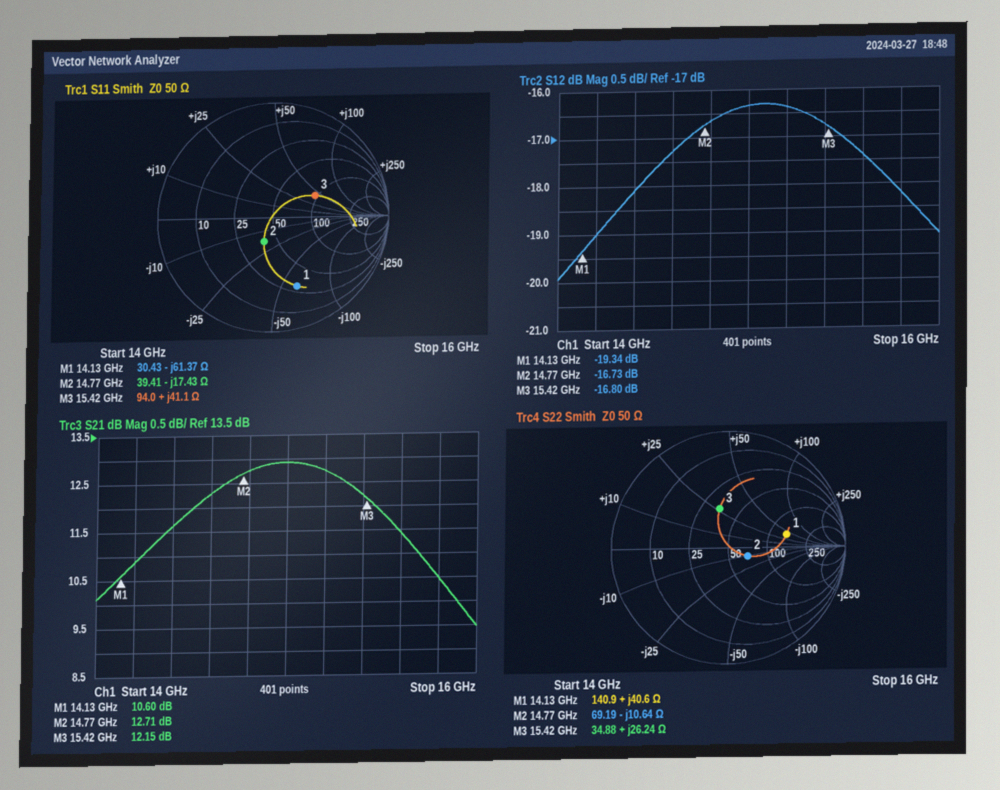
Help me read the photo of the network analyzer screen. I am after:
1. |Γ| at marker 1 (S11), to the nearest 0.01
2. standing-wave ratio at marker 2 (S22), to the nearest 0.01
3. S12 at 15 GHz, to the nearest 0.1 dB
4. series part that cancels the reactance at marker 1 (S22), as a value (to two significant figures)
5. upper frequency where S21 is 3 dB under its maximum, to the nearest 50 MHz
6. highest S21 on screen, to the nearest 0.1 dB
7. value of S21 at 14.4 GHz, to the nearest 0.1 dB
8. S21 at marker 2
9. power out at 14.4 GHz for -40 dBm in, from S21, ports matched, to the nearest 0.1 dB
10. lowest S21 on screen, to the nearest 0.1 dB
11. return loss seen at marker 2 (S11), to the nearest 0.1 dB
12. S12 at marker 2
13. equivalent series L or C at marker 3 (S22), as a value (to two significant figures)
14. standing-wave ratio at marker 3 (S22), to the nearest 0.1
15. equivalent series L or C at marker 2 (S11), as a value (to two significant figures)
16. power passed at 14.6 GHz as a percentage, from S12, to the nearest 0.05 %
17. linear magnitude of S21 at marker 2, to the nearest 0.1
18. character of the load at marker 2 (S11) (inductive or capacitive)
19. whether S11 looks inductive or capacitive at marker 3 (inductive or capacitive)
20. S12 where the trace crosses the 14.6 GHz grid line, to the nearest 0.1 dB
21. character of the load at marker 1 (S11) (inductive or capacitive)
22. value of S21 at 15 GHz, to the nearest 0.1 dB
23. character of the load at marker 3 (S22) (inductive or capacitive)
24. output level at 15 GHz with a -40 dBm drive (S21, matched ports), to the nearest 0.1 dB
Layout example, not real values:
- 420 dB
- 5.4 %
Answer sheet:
- 0.64
- 1.45
- -16.3 dB
- 280 fF
- 15.90 GHz
- 12.9 dB
- 11.6 dB
- 12.71 dB
- -28.4 dBm
- 9.5 dB
- 13.0 dB
- -16.73 dB
- 270 pH
- 2.0
- 620 fF
- 1.85 %
- 4.3
- capacitive
- inductive
- -17.3 dB
- capacitive
- 12.9 dB
- inductive
- -27.1 dBm
